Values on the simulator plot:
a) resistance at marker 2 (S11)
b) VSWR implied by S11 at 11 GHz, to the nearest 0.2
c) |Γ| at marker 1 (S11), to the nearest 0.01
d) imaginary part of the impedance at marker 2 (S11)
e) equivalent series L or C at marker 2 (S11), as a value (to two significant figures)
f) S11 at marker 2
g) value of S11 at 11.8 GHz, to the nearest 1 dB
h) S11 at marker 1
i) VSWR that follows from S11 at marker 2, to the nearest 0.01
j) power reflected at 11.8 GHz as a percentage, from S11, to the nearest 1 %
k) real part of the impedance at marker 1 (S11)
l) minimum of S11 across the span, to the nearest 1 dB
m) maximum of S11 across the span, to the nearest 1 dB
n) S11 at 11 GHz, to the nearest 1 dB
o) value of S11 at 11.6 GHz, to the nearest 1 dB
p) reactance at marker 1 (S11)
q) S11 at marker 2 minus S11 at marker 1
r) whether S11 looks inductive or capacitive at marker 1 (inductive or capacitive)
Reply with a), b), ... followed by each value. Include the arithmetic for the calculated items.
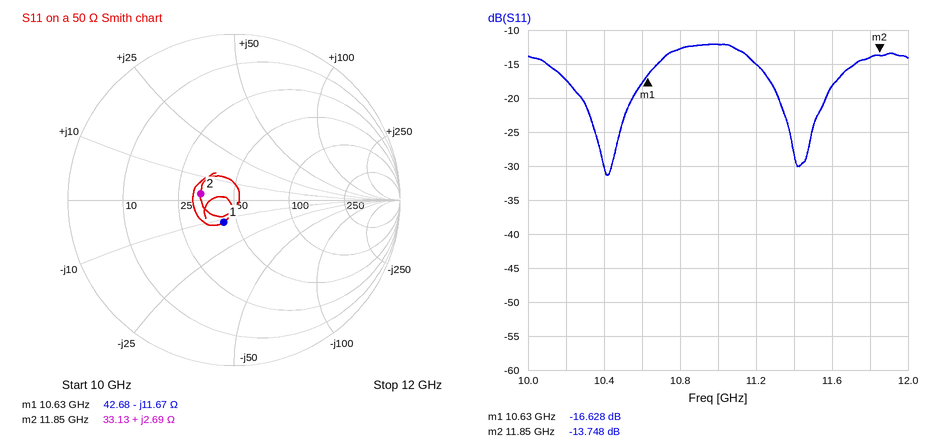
a) 33.13 Ω
b) |Γ| = 10^(-12/20) = 0.2512; VSWR = (1 + 0.2512)/(1 − 0.2512) ≈ 1.67, so 1.6 to the nearest 0.2
c) 0.15
d) +2.69 Ω
e) L = 2.69 Ω/(2π × 11.85 GHz) ≈ 36 pH
f) -13.748 dB
g) -14 dB
h) -16.628 dB
i) (1 + 0.2054)/(1 − 0.2054) ≈ 1.52
j) 10^(-14/10) ≈ 4 %
k) 42.68 Ω
l) -31 dB
m) -12 dB
n) -12 dB
o) -18 dB
p) -11.67 Ω
q) -13.748 − (-16.628) = 2.880 dB
r) capacitive
